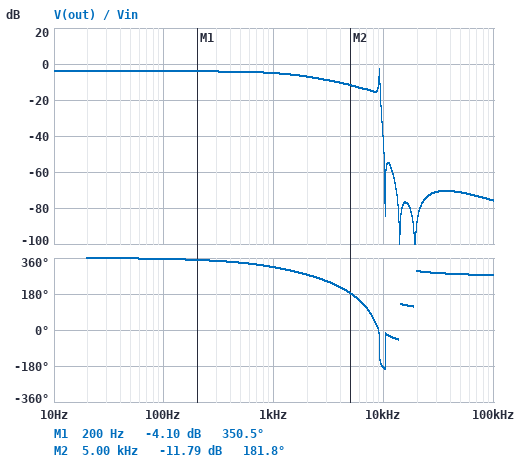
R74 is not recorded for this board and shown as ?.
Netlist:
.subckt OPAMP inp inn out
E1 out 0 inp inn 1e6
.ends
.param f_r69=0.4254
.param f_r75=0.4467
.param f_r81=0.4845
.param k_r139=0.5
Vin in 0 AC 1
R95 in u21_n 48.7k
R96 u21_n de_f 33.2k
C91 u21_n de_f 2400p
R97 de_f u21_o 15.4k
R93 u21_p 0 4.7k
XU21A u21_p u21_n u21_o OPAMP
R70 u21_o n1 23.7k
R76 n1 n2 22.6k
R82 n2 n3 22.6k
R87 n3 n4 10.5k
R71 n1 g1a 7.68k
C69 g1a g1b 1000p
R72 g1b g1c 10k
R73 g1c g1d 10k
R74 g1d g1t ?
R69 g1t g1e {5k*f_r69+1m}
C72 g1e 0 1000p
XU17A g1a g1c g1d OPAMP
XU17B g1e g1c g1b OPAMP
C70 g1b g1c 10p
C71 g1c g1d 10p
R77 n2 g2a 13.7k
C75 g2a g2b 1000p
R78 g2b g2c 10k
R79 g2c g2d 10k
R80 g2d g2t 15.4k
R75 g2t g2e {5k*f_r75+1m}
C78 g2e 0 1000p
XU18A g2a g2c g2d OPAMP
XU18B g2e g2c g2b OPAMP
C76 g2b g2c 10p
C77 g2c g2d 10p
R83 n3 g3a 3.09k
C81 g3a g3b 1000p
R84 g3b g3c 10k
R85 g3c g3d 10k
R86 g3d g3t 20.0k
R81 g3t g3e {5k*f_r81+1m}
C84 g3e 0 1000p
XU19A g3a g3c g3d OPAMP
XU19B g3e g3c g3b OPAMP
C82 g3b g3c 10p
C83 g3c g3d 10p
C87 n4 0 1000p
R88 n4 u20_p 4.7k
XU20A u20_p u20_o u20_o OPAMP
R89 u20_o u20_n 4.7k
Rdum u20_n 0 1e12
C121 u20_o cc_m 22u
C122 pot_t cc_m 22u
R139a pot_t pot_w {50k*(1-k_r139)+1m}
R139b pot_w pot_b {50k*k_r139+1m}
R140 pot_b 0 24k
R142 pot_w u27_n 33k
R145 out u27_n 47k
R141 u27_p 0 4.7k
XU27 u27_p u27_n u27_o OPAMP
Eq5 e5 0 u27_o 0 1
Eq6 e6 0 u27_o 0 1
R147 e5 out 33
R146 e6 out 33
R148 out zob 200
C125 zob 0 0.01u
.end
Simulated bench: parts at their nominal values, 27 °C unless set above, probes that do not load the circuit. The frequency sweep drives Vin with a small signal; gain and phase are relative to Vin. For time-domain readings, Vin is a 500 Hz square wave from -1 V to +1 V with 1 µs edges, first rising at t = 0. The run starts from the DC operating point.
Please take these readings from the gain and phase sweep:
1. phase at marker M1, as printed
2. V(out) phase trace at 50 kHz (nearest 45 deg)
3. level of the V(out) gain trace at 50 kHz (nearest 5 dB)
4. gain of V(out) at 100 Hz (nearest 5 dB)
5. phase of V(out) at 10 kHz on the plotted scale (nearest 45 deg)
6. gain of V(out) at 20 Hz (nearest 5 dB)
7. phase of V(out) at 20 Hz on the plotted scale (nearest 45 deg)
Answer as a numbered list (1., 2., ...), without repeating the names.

1. 350.5 deg
2. 270 deg
3. -70 dB
4. -5 dB
5. -180 deg
6. -5 dB
7. 360 deg
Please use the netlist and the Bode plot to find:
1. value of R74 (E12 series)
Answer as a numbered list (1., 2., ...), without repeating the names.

1. 15 kΩ
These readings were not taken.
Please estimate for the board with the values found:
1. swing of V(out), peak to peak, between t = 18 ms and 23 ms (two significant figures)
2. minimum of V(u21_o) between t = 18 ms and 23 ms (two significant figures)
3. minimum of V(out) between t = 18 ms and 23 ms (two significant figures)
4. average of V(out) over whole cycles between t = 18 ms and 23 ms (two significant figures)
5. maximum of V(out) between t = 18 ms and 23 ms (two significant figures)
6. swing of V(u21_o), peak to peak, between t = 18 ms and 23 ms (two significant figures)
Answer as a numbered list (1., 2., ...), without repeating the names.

1. 1.3 V
2. -1.0 V
3. -35 mV
4. 600 mV
5. 1.2 V
6. 2.0 V
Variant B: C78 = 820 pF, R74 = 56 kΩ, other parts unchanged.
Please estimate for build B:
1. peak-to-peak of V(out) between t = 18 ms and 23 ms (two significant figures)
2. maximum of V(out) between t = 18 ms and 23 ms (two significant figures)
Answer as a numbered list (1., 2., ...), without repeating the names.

1. 1.4 V
2. 1.3 V
